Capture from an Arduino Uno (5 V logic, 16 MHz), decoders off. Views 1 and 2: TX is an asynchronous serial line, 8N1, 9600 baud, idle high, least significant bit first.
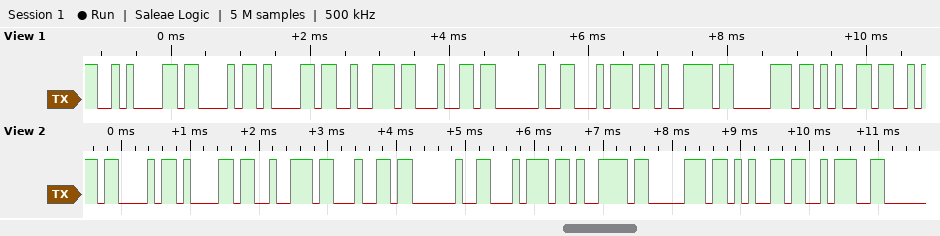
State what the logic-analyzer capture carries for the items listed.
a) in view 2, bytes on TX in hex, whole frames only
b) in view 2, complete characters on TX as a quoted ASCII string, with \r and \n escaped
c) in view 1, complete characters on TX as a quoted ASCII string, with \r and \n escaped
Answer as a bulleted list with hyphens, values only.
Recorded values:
- 43 61 72 64 20 74 79 70 65 3A
- "Card type:"
- "\nCard type"
